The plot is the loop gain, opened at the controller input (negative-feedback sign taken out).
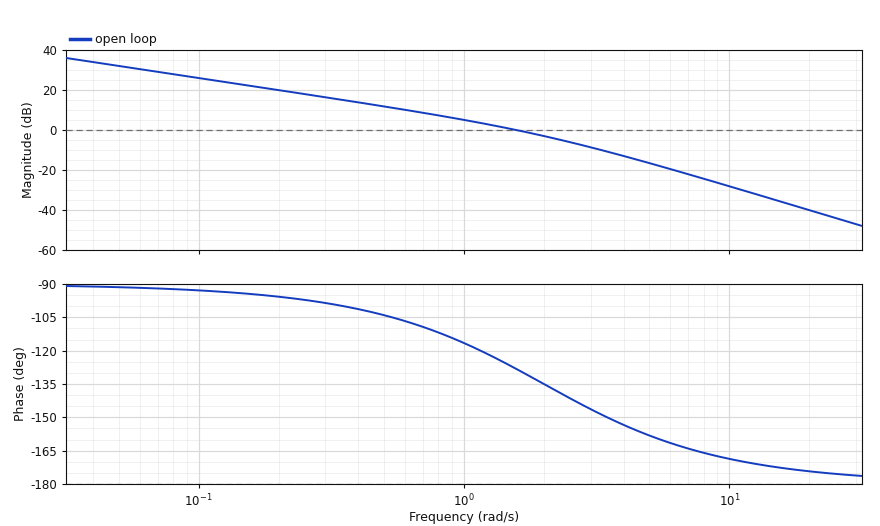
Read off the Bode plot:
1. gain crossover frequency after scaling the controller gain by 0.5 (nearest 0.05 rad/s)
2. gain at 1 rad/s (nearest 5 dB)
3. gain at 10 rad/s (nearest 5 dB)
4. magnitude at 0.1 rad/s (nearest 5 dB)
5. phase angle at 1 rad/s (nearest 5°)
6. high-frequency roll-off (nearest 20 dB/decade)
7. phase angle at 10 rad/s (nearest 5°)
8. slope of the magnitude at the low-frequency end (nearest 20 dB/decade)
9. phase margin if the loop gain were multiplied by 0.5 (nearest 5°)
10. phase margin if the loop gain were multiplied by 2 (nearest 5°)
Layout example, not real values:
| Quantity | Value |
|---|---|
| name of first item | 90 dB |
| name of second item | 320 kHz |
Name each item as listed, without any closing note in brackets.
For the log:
| Quantity | Value |
|---|---|
| gain crossover frequency after scaling the controller gain by 0.5 | 0.90 rad/s |
| gain at 1 rad/s | 5 dB |
| gain at 10 rad/s | -30 dB |
| magnitude at 0.1 rad/s | 25 dB |
| phase angle at 1 rad/s | -115° |
| high-frequency roll-off | -40 dB/decade |
| phase angle at 10 rad/s | -170° |
| slope of the magnitude at the low-frequency end | -20 dB/decade |
| phase margin if the loop gain were multiplied by 0.5 | 65° |
| phase margin if the loop gain were multiplied by 2 | 40° |
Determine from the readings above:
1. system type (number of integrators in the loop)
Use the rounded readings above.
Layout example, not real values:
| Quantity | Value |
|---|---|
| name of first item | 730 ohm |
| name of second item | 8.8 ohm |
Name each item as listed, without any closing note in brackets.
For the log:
| Quantity | Value |
|---|---|
| system type | 1 |
